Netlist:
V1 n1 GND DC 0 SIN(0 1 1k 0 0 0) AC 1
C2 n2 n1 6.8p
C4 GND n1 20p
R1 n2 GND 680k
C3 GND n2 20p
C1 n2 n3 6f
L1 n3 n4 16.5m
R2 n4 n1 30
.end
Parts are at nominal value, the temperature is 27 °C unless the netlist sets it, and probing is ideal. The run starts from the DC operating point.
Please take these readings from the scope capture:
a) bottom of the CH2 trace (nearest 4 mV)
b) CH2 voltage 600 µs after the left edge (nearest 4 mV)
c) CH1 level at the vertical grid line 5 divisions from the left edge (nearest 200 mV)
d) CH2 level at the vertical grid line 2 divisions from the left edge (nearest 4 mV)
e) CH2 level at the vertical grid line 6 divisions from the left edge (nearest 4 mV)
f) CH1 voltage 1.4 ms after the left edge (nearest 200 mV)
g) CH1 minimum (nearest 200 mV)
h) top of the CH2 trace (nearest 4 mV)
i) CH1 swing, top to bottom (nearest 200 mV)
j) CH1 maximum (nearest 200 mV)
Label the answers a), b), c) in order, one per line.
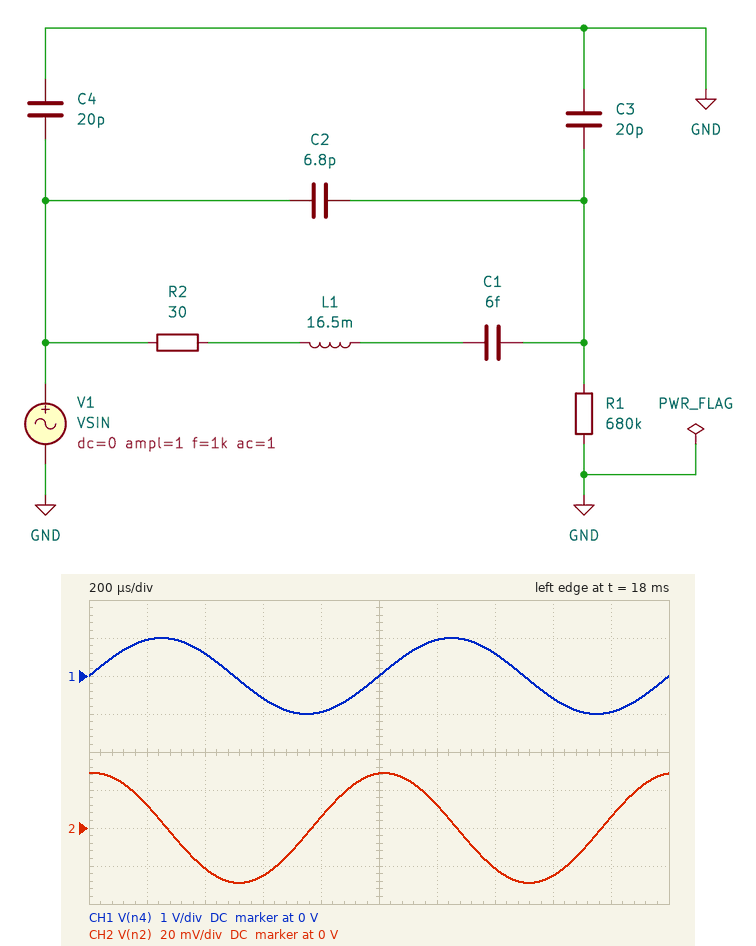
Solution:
a) -28 mV
b) -24 mV
c) 0 V
d) -20 mV
e) 12 mV
f) 600 mV
g) -1.0 V
h) 28 mV
i) 2.0 V
j) 1.0 V
